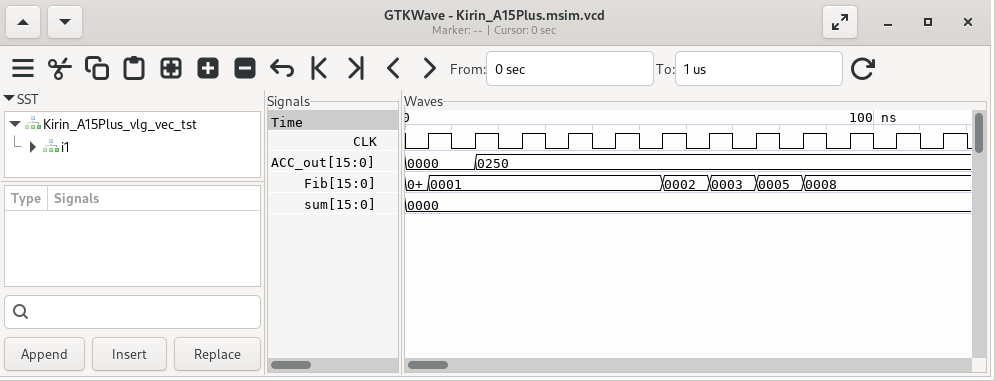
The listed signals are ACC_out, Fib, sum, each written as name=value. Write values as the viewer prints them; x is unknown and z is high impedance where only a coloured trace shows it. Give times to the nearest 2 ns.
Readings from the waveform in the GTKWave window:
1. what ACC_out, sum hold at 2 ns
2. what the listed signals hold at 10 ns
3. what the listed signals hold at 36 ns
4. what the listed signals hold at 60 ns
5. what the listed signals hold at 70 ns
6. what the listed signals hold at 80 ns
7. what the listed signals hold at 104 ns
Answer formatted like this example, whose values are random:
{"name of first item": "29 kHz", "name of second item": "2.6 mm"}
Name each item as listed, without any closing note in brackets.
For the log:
{"what ACC_out, sum hold at 2 ns": "ACC_out=0000, sum=0000", "what the listed signals hold at 10 ns": "ACC_out=0000, Fib=0001, sum=0000", "what the listed signals hold at 36 ns": "ACC_out=0250, Fib=0001, sum=0000", "what the listed signals hold at 60 ns": "ACC_out=0250, Fib=0002, sum=0000", "what the listed signals hold at 70 ns": "ACC_out=0250, Fib=0003, sum=0000", "what the listed signals hold at 80 ns": "ACC_out=0250, Fib=0005, sum=0000", "what the listed signals hold at 104 ns": "ACC_out=0250, Fib=0008, sum=0000"}
